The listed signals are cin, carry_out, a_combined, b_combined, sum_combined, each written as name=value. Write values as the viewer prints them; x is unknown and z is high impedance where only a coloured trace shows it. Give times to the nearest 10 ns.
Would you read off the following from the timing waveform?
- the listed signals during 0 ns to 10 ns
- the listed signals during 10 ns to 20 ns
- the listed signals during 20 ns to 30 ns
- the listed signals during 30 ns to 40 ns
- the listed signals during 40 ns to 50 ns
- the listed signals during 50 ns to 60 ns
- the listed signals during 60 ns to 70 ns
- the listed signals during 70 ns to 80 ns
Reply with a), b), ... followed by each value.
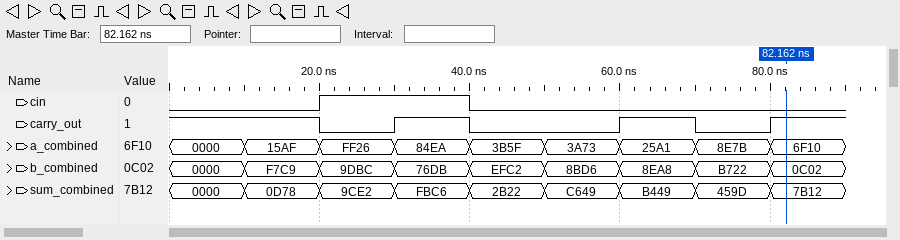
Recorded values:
a) cin=0, carry_out=1, a_combined=0000, b_combined=0000, sum_combined=0000
b) cin=0, carry_out=1, a_combined=15AF, b_combined=F7C9, sum_combined=0D78
c) cin=1, carry_out=0, a_combined=FF26, b_combined=9DBC, sum_combined=9CE2
d) cin=1, carry_out=1, a_combined=84EA, b_combined=76DB, sum_combined=FBC6
e) cin=0, carry_out=0, a_combined=3B5F, b_combined=EFC2, sum_combined=2B22
f) cin=0, carry_out=0, a_combined=3A73, b_combined=8BD6, sum_combined=C649
g) cin=0, carry_out=1, a_combined=25A1, b_combined=8EA8, sum_combined=B449
h) cin=0, carry_out=0, a_combined=8E7B, b_combined=B722, sum_combined=459D
